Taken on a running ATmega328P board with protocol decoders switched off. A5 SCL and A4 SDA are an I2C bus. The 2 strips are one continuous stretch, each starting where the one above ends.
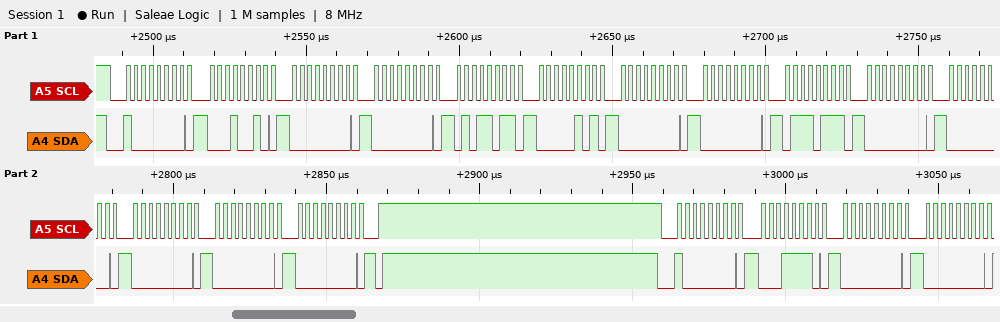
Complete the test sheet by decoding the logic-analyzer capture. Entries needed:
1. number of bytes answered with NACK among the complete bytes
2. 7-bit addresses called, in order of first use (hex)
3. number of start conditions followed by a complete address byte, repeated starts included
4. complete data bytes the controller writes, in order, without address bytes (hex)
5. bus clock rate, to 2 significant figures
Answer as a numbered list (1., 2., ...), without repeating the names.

1. 0
2. 0x40
3. 2
4. 12 00 00 5B 05 00 00 77 00 00 00 00 00 1E 00 00
5. 400 kHz
